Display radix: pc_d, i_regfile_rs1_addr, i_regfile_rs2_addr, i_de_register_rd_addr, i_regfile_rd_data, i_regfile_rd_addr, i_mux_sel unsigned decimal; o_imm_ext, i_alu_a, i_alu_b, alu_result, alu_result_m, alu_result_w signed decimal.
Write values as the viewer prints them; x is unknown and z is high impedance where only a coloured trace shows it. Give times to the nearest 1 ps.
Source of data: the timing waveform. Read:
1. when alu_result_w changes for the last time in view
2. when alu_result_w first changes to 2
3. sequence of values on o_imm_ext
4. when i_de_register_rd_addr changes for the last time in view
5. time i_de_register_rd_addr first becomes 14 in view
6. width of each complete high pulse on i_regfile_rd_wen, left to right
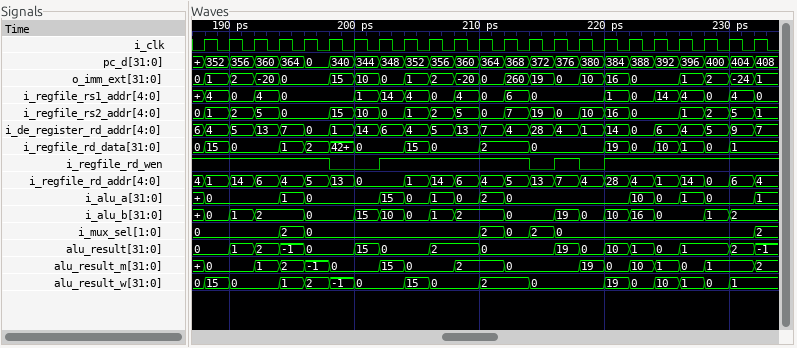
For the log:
230 ps
196 ps
0, 1, 2, -20, 0, 15, 10, 0, 1, 2, -20, 0, 260, 19, 0, 10, 16, 0, 1, 2, -24, 1
232 ps
200 ps
12 ps, 2 ps
